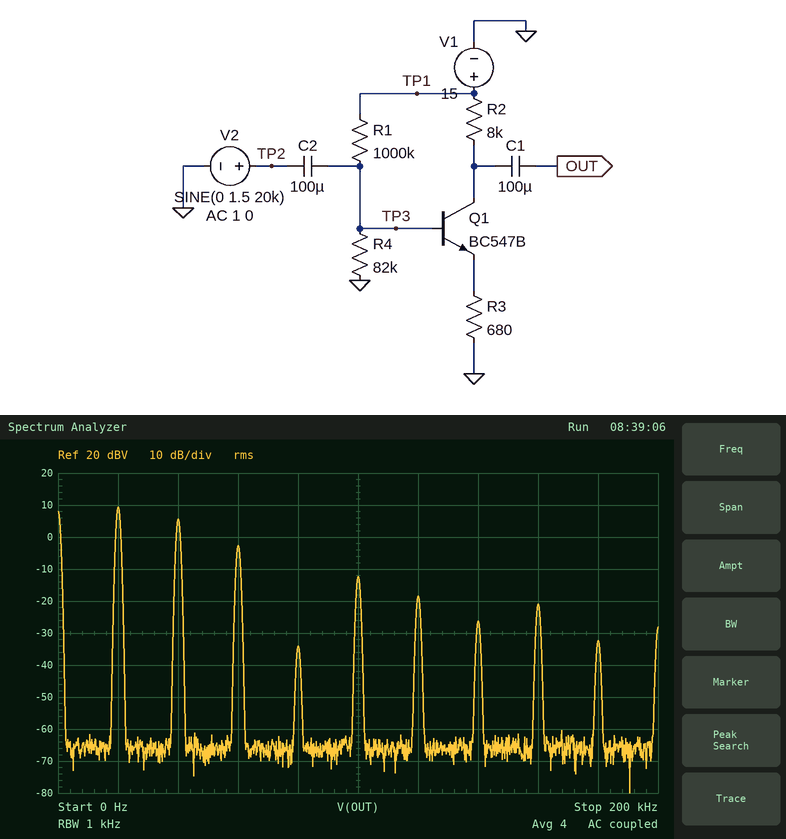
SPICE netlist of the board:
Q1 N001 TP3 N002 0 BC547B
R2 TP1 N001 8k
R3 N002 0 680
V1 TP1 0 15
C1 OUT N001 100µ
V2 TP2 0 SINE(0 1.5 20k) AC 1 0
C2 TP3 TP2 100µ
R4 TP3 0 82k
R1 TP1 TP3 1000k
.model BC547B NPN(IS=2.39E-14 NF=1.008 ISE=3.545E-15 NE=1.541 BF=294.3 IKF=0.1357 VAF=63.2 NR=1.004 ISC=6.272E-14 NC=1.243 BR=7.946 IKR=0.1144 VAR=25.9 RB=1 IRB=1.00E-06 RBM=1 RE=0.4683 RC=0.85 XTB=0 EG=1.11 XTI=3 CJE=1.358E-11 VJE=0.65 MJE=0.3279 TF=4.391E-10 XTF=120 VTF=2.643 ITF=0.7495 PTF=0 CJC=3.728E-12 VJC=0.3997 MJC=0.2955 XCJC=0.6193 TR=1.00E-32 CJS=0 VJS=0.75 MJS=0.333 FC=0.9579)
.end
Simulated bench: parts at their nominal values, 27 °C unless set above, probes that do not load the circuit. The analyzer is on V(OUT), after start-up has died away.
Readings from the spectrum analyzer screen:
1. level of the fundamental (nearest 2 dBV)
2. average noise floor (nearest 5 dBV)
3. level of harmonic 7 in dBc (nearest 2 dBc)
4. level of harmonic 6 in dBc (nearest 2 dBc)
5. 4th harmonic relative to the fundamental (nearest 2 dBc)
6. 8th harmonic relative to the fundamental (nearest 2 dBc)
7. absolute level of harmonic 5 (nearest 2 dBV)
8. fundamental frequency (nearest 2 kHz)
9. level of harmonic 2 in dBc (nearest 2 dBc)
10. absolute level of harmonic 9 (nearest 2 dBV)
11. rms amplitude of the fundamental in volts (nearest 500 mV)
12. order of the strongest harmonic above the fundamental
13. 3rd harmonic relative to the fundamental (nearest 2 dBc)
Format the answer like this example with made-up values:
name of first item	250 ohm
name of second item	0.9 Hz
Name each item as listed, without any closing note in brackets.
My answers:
level of the fundamental	10 dBV
average noise floor	-65 dBV
level of harmonic 7 in dBc	-36 dBc
level of harmonic 6 in dBc	-28 dBc
4th harmonic relative to the fundamental	-44 dBc
8th harmonic relative to the fundamental	-30 dBc
absolute level of harmonic 5	-12 dBV
fundamental frequency	20 kHz
level of harmonic 2 in dBc	-4 dBc
absolute level of harmonic 9	-32 dBV
rms amplitude of the fundamental in volts	3.0 V
order of the strongest harmonic above the fundamental	2
3rd harmonic relative to the fundamental	-12 dBc
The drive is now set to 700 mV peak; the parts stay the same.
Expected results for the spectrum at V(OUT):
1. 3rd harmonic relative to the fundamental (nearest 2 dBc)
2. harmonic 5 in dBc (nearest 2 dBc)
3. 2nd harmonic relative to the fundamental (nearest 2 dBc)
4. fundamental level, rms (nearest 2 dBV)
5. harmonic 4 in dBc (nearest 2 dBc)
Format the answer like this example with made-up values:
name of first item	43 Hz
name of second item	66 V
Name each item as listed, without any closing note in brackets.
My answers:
3rd harmonic relative to the fundamental	-4 dBc
harmonic 5 in dBc	-14 dBc
2nd harmonic relative to the fundamental	-2 dBc
fundamental level, rms	-12 dBV
harmonic 4 in dBc	-8 dBc
